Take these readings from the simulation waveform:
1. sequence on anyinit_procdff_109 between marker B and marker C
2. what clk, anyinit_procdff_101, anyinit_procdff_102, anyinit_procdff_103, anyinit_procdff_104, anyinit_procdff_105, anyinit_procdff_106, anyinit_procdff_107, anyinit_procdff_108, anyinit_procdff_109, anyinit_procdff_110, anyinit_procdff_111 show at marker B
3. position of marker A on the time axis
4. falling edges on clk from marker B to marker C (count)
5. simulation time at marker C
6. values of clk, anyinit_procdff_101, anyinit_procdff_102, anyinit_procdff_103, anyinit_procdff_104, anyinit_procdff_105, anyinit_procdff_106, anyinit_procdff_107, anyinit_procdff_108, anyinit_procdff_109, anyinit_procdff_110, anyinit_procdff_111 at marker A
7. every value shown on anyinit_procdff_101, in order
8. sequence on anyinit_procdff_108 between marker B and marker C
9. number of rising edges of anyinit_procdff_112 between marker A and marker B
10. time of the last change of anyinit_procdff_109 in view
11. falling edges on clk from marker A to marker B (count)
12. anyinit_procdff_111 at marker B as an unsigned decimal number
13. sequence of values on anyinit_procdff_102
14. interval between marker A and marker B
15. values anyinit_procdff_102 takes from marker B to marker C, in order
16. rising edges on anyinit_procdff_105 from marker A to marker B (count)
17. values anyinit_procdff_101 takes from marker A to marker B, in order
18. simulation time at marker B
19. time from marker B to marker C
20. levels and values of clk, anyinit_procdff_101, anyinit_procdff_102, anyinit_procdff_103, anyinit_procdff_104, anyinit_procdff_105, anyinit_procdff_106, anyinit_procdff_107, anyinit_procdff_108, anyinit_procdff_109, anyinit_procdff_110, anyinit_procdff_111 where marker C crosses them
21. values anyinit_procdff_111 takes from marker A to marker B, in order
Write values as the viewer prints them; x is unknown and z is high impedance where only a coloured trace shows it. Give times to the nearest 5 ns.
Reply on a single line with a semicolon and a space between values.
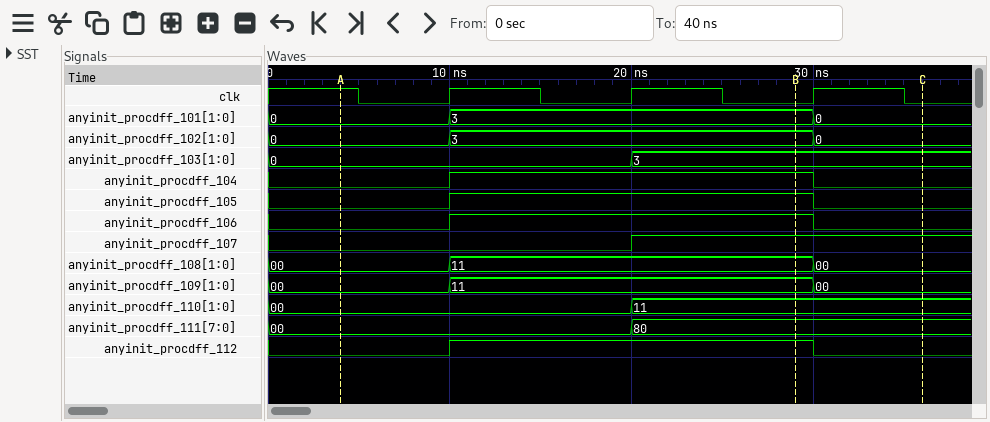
11, 00; clk=0, anyinit_procdff_101=3, anyinit_procdff_102=3, anyinit_procdff_103=3, anyinit_procdff_104=1, anyinit_procdff_105=1, anyinit_procdff_106=1, anyinit_procdff_107=1, anyinit_procdff_108=11, anyinit_procdff_109=11, anyinit_procdff_110=11, anyinit_procdff_111=80; 5 ns; 1; 35 ns; clk=1, anyinit_procdff_101=0, anyinit_procdff_102=0, anyinit_procdff_103=0, anyinit_procdff_104=0, anyinit_procdff_105=0, anyinit_procdff_106=0, anyinit_procdff_107=0, anyinit_procdff_108=00, anyinit_procdff_109=00, anyinit_procdff_110=00, anyinit_procdff_111=00; 0, 3, 0; 11, 00; 1; 30 ns; 3; 128; 0, 3, 0; 25 ns; 3, 0; 1; 0, 3; 30 ns; 5 ns; clk=0, anyinit_procdff_101=0, anyinit_procdff_102=0, anyinit_procdff_103=3, anyinit_procdff_104=0, anyinit_procdff_105=0, anyinit_procdff_106=0, anyinit_procdff_107=1, anyinit_procdff_108=00, anyinit_procdff_109=00, anyinit_procdff_110=11, anyinit_procdff_111=80; 00, 80
